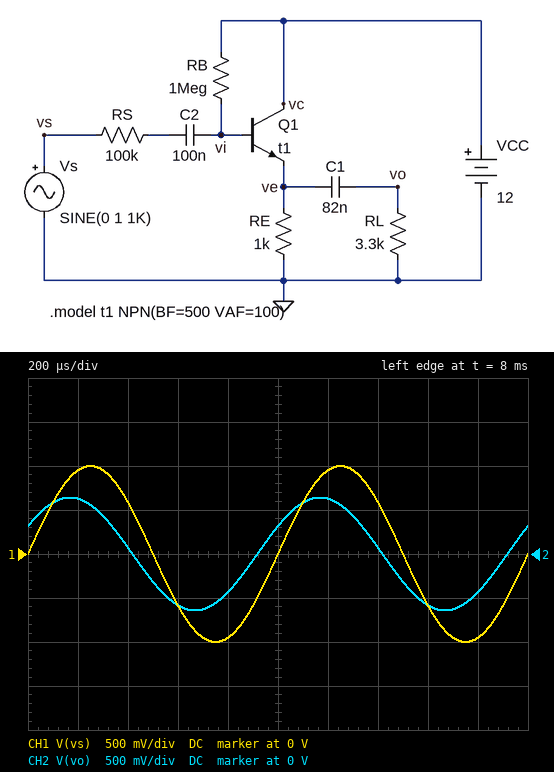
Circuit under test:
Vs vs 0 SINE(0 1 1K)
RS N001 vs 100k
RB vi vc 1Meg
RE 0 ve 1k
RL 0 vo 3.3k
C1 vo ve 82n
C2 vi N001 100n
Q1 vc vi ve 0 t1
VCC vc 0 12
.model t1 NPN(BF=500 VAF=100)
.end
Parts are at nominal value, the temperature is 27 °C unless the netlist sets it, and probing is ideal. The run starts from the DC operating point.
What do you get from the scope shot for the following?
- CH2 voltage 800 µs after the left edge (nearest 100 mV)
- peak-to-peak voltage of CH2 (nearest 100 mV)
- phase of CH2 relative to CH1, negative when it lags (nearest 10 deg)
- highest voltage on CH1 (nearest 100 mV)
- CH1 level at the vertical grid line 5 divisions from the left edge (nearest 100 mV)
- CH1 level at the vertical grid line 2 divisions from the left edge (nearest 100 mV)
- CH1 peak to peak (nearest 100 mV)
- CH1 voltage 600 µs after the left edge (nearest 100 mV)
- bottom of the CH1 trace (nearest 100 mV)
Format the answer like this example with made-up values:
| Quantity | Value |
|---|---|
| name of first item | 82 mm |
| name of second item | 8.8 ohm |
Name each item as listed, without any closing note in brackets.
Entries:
| Quantity | Value |
|---|---|
| CH2 voltage 800 µs after the left edge | -400 mV |
| peak-to-peak voltage of CH2 | 1.3 V |
| phase of CH2 relative to CH1, negative when it lags | 30 deg |
| highest voltage on CH1 | 1.0 V |
| CH1 level at the vertical grid line 5 divisions from the left edge | 0 V |
| CH1 level at the vertical grid line 2 divisions from the left edge | 600 mV |
| CH1 peak to peak | 2.0 V |
| CH1 voltage 600 µs after the left edge | -600 mV |
| bottom of the CH1 trace | -1.0 V |
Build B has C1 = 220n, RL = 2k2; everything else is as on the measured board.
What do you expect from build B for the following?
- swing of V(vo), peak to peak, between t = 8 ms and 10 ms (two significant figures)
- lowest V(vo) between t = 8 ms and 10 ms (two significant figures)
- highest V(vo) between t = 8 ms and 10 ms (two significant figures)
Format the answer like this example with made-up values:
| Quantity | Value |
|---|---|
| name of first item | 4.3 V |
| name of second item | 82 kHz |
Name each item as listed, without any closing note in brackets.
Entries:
| Quantity | Value |
|---|---|
| swing of V(vo), peak to peak, between t = 8 ms and 10 ms | 1.4 V |
| lowest V(vo) between t = 8 ms and 10 ms | -690 mV |
| highest V(vo) between t = 8 ms and 10 ms | 690 mV |
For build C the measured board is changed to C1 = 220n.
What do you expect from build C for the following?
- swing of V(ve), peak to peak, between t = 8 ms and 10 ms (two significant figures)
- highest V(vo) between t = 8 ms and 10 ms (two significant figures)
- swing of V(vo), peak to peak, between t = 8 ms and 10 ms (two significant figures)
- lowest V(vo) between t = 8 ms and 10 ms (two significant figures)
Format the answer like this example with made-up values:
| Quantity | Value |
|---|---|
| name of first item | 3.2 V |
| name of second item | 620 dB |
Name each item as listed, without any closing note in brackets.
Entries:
| Quantity | Value |
|---|---|
| swing of V(ve), peak to peak, between t = 8 ms and 10 ms | 1.5 V |
| highest V(vo) between t = 8 ms and 10 ms | 720 mV |
| swing of V(vo), peak to peak, between t = 8 ms and 10 ms | 1.4 V |
| lowest V(vo) between t = 8 ms and 10 ms | -720 mV |
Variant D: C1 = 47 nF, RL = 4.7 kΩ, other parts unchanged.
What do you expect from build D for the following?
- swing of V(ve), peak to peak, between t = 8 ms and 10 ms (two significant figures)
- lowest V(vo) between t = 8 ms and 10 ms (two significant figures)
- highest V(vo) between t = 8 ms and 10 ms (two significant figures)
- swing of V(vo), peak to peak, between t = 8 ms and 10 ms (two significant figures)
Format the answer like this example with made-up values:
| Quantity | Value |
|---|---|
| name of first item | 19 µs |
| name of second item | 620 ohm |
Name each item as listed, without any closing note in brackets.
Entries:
| Quantity | Value |
|---|---|
| swing of V(ve), peak to peak, between t = 8 ms and 10 ms | 1.5 V |
| lowest V(vo) between t = 8 ms and 10 ms | -610 mV |
| highest V(vo) between t = 8 ms and 10 ms | 610 mV |
| swing of V(vo), peak to peak, between t = 8 ms and 10 ms | 1.2 V |
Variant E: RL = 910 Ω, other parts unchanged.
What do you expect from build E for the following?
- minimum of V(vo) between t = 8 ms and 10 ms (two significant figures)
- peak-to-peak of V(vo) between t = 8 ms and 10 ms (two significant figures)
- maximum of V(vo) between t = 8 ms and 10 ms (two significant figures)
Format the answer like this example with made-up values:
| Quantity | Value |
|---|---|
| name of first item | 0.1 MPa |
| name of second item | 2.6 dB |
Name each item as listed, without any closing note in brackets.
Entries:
| Quantity | Value |
|---|---|
| minimum of V(vo) between t = 8 ms and 10 ms | -320 mV |
| peak-to-peak of V(vo) between t = 8 ms and 10 ms | 630 mV |
| maximum of V(vo) between t = 8 ms and 10 ms | 320 mV |
